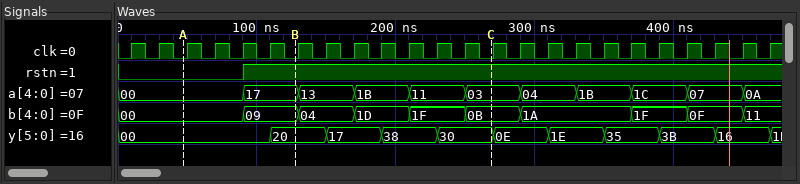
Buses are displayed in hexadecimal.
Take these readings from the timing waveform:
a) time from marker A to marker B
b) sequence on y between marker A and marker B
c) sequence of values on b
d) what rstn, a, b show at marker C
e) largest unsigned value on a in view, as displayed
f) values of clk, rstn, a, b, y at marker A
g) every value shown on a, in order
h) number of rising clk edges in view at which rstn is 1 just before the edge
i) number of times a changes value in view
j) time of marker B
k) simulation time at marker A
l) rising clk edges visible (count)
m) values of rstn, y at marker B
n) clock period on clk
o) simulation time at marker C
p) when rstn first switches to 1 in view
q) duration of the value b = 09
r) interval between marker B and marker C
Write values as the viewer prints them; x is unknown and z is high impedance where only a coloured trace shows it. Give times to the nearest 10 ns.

80 ns
00, 20
00, 09, 04, 1D, 1F, 0B, 1A, 1F, 0F, 11
rstn=1, a=03, b=0B
1C
clk=0, rstn=0, a=00, b=00, y=00
00, 17, 13, 1B, 11, 03, 04, 1B, 1C, 07, 0A
19
10
130 ns
50 ns
24
rstn=1, y=20
20 ns
270 ns
90 ns
40 ns
140 ns
